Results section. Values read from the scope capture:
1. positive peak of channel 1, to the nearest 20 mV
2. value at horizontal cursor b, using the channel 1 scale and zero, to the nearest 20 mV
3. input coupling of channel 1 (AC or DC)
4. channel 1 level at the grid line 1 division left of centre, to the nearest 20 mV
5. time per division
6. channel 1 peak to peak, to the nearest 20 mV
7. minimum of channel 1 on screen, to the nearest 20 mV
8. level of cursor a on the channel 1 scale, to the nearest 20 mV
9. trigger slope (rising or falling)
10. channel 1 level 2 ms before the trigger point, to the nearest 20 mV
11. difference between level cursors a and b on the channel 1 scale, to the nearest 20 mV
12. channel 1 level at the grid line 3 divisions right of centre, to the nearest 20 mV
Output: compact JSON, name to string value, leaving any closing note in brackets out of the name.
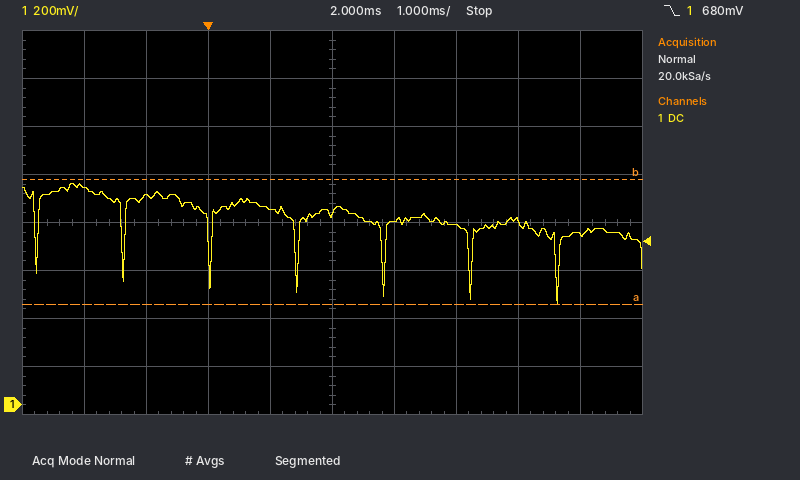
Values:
{"positive peak of channel 1, to the nearest 20 mV": "920 mV", "value at horizontal cursor b, using the channel 1 scale and zero, to the nearest 20 mV": "940 mV", "input coupling of channel 1": "DC", "channel 1 level at the grid line 1 division left of centre, to the nearest 20 mV": "820 mV", "time per division": "1 ms", "channel 1 peak to peak, to the nearest 20 mV": "500 mV", "minimum of channel 1 on screen, to the nearest 20 mV": "420 mV", "level of cursor a on the channel 1 scale, to the nearest 20 mV": "420 mV", "trigger slope": "falling", "channel 1 level 2 ms before the trigger point, to the nearest 20 mV": "900 mV", "difference between level cursors a and b on the channel 1 scale, to the nearest 20 mV": "520 mV", "channel 1 level at the grid line 3 divisions right of centre, to the nearest 20 mV": "760 mV"}
